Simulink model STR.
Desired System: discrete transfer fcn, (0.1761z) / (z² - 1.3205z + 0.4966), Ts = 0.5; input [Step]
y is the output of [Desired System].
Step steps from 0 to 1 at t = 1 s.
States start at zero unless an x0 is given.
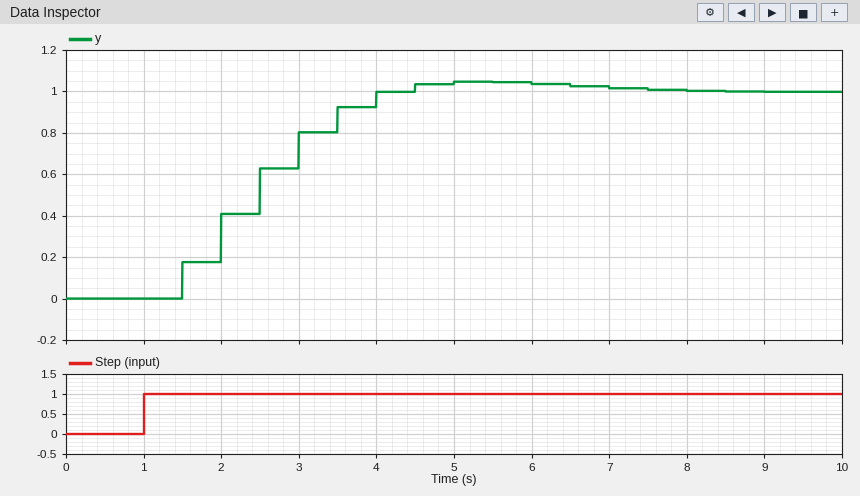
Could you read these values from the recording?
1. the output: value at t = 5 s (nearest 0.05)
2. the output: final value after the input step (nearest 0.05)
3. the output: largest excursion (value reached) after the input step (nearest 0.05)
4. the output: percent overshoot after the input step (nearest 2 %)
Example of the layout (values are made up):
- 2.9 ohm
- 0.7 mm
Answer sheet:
- 1.05
- 1.00
- 1.05
- 4 %
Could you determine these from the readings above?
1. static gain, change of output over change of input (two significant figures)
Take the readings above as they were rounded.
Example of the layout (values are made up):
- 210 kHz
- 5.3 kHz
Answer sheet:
- 1.0
